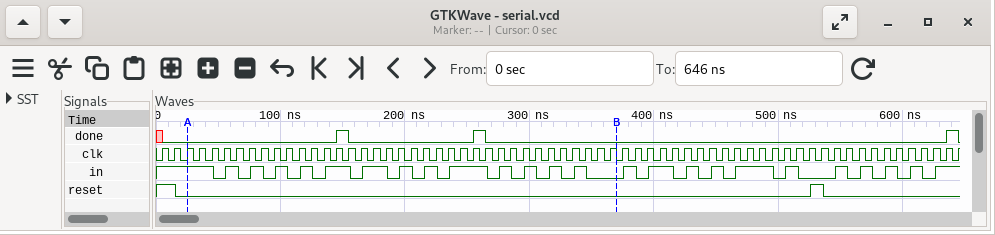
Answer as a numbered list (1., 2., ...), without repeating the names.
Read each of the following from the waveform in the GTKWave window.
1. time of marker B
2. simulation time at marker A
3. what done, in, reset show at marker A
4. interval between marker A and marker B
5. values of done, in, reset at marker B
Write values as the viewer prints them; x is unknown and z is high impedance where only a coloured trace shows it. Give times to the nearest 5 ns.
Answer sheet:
1. 370 ns
2. 25 ns
3. done=0, in=1, reset=0
4. 345 ns
5. done=0, in=0, reset=0
